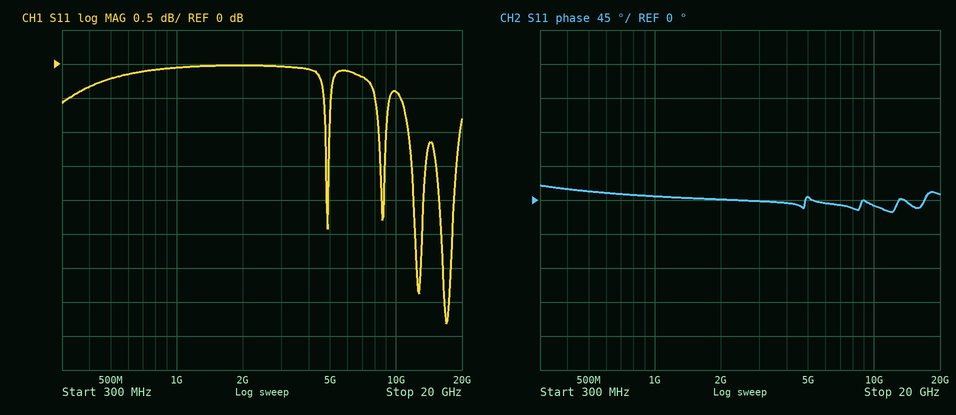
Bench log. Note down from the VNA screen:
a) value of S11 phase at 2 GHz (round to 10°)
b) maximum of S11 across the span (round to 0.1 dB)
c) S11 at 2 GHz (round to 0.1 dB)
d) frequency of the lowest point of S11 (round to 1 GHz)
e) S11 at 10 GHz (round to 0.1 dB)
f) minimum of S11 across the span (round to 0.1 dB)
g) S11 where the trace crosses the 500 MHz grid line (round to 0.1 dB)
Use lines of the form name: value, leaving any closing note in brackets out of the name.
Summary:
value of S11 phase at 2 GHz: 0°
maximum of S11 across the span: 0.0 dB
S11 at 2 GHz: 0.0 dB
frequency of the lowest point of S11: 17 GHz
S11 at 10 GHz: -0.4 dB
minimum of S11 across the span: -3.8 dB
S11 where the trace crosses the 500 MHz grid line: -0.2 dB
